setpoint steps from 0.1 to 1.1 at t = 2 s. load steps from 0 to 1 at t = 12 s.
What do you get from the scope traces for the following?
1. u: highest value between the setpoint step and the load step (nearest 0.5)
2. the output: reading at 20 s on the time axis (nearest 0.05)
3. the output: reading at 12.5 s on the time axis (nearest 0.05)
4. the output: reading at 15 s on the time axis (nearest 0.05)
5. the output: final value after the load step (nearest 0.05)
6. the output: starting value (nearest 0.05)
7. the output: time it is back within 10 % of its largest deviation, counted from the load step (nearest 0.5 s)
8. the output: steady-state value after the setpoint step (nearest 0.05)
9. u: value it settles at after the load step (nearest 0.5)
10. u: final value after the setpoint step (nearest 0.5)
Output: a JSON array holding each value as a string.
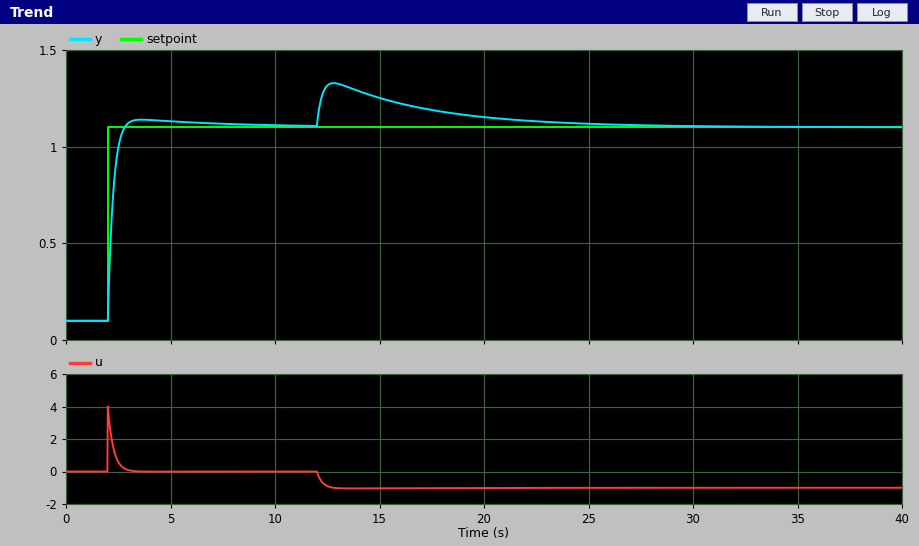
["4.0", "1.15", "1.30", "1.25", "1.10", "0.10", "12.0 s", "1.10", "-1.0", "0.0"]
